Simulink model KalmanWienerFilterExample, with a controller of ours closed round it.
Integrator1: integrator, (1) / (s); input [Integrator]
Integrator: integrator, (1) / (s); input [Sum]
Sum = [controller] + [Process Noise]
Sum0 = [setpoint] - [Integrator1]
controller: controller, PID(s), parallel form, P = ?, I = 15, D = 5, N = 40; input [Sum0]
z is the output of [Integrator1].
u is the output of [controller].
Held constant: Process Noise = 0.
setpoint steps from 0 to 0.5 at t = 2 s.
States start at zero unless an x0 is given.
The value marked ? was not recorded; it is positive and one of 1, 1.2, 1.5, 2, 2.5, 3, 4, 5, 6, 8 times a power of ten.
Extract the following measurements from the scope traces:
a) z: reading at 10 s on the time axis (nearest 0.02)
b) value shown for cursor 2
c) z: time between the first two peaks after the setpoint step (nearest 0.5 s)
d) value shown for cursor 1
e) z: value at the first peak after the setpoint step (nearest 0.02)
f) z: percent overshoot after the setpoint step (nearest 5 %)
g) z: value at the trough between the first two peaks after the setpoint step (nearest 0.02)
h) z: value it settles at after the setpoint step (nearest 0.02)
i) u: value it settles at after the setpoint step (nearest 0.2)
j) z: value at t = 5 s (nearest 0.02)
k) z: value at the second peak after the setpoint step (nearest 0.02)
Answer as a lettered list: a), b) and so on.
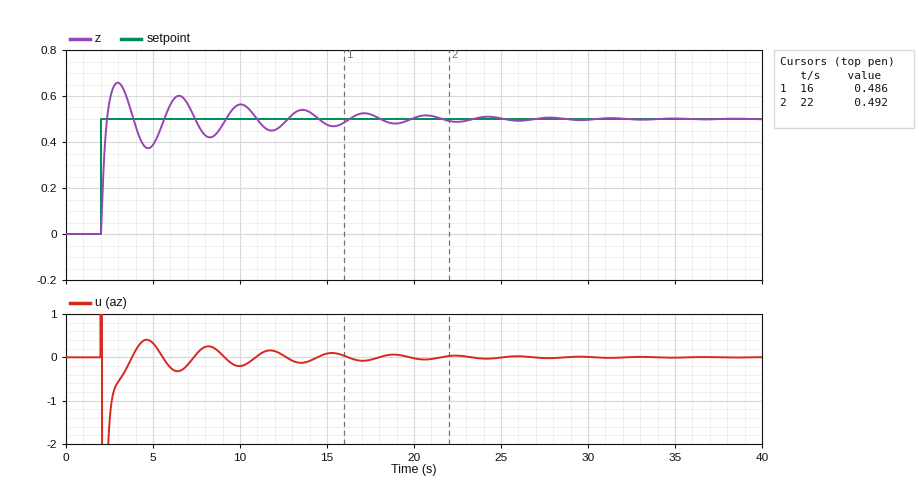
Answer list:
a) 0.56
b) 0.492
c) 3.5 s
d) 0.486
e) 0.66
f) 30 %
g) 0.38
h) 0.50
i) 0.0
j) 0.38
k) 0.60
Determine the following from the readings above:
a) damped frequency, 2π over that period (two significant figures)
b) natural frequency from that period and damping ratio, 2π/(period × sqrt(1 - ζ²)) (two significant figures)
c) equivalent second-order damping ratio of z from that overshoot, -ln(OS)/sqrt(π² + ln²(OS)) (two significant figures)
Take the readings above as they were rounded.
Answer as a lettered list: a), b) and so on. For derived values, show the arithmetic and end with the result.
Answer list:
a) 2π / 3.5 = 1.8 rad/s
b) 2π / (3.5 × sqrt(1 - 0.36²)) = 1.9 rad/s
c) ln(0.3) = -1.204; 1.204 / sqrt(9.870 + 1.450) = 0.36
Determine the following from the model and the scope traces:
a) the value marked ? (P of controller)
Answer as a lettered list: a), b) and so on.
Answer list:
a) 4
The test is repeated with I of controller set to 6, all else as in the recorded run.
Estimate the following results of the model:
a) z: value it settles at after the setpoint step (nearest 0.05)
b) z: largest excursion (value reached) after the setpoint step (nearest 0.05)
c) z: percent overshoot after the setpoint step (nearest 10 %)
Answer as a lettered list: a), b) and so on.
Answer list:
a) 0.50
b) 0.60
c) 20 %
